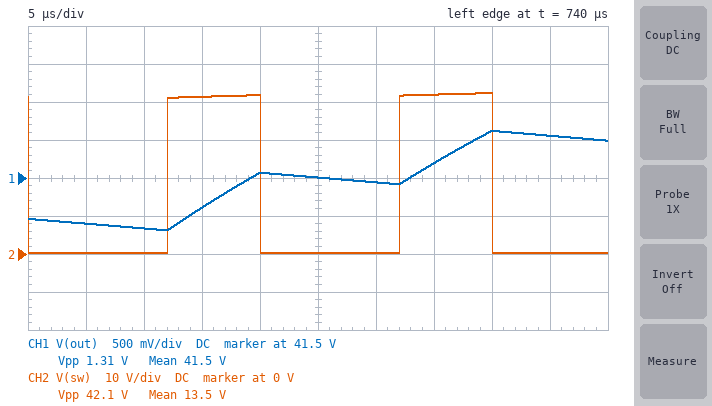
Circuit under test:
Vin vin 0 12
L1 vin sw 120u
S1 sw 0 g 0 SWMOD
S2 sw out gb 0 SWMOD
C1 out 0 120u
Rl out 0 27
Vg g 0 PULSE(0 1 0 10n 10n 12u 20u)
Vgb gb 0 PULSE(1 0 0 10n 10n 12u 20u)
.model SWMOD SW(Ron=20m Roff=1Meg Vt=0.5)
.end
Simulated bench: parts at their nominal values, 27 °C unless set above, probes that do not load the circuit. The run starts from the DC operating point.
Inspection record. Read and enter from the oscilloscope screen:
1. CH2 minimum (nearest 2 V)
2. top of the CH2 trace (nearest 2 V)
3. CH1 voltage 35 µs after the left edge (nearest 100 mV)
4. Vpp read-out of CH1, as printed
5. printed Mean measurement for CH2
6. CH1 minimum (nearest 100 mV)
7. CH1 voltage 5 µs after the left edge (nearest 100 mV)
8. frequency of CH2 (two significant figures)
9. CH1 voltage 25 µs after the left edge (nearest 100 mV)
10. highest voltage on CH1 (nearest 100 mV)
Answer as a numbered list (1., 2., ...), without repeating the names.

1. 0 V
2. 42 V
3. 41.7 V
4. 1.31 V
5. 13.5 V
6. 40.8 V
7. 40.9 V
8. 50 kHz
9. 41.5 V
10. 42.1 V
